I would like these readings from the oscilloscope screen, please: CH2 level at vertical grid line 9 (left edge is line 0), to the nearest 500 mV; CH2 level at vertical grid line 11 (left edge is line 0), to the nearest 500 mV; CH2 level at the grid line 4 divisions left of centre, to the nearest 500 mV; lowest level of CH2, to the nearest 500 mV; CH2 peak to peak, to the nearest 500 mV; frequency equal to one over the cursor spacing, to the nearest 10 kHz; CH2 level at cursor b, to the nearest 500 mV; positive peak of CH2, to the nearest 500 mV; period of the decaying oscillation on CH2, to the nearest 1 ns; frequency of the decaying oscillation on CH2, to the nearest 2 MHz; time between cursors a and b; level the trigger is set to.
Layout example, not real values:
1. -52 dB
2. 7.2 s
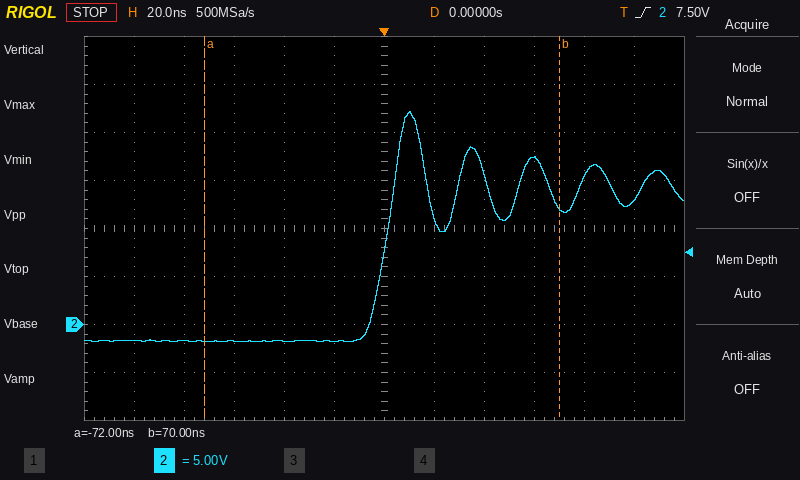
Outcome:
1. 17.5 V
2. 13.0 V
3. -1.5 V
4. -2.0 V
5. 24.0 V
6. 7.04 MHz
7. 12.0 V
8. 22.0 V
9. 25 ns
10. 40 MHz
11. 142 ns
12. 7.50 V
